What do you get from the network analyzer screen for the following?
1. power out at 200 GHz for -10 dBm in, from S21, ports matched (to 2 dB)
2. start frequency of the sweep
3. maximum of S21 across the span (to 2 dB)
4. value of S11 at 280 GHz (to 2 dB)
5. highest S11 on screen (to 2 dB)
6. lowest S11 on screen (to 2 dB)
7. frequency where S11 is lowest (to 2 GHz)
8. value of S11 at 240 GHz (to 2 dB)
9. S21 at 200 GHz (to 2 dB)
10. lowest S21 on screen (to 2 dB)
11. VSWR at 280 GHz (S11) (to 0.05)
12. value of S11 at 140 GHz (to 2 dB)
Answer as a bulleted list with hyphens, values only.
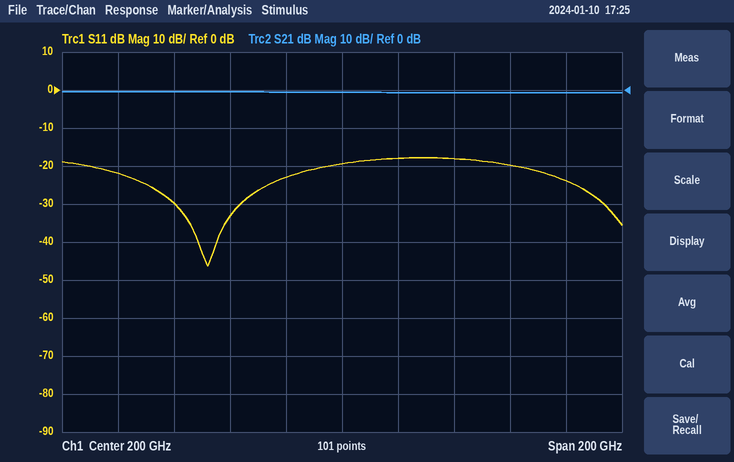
- -10 dBm
- 100 GHz
- 0 dB
- -24 dB
- -18 dB
- -46 dB
- 152 GHz
- -18 dB
- 0 dB
- 0 dB
- 1.15
- -30 dB
